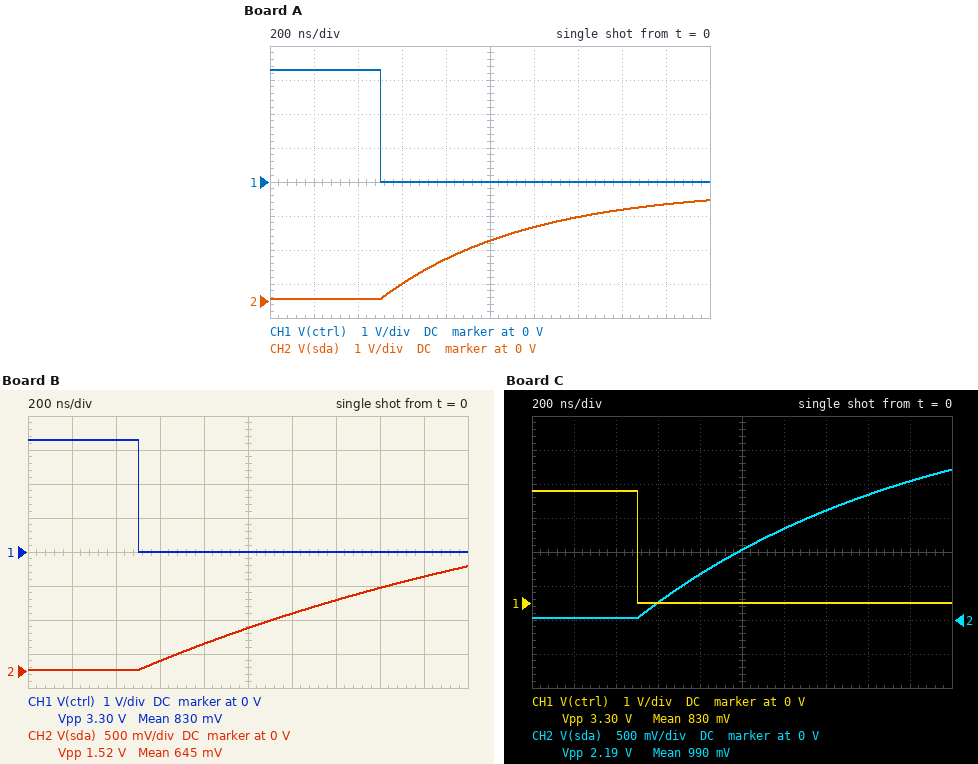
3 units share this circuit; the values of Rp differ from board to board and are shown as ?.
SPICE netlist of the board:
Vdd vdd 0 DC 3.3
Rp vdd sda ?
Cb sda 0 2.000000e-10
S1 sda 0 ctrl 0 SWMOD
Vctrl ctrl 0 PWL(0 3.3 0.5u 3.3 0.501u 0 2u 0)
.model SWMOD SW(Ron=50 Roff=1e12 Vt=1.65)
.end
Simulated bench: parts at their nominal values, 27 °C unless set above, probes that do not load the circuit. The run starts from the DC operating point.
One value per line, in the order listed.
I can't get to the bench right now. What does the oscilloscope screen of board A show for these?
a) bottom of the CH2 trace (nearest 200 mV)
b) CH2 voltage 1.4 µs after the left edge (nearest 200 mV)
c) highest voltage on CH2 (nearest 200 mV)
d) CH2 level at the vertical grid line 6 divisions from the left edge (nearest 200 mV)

0 V
2.4 V
3.0 V
2.2 V
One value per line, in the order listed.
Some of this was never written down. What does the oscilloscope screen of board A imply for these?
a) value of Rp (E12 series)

3.3 kΩ
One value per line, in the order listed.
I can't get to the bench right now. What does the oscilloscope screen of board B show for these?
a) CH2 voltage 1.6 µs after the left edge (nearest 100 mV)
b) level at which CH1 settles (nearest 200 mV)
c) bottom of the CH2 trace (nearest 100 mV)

1.2 V
0 V
0 V
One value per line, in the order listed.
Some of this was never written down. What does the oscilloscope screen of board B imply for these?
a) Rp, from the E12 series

12 kΩ
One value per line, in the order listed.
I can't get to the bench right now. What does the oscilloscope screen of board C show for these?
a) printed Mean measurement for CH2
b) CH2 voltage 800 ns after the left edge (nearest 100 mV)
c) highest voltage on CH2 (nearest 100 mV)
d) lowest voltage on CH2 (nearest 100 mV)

990 mV
700 mV
2.2 V
0 V
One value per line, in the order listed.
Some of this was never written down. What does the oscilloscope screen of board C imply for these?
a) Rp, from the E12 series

6.8 kΩ
